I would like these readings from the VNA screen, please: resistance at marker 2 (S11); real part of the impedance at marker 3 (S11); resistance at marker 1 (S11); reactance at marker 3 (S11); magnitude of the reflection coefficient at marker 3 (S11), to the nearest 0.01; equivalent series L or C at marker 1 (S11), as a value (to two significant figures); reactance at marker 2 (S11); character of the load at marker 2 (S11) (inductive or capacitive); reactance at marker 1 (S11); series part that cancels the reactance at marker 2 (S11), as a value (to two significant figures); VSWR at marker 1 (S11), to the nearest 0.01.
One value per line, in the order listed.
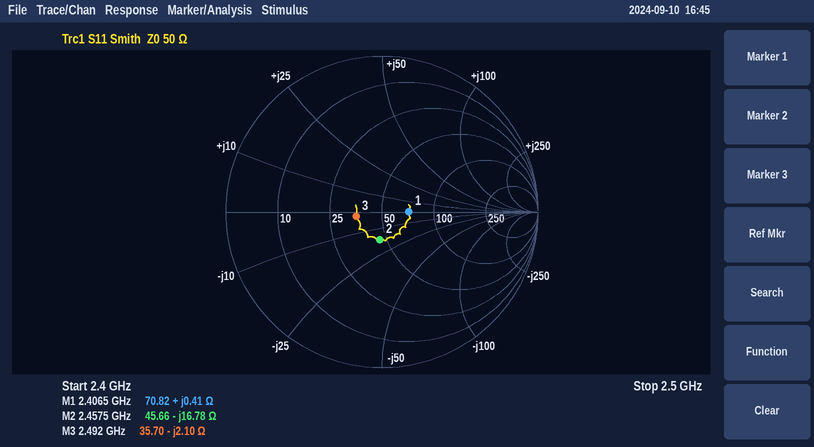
45.66 Ω
35.70 Ω
70.82 Ω
-2.10 Ω
0.17
27 pH
-16.78 Ω
capacitive
+0.41 Ω
1.1 nH
1.42
